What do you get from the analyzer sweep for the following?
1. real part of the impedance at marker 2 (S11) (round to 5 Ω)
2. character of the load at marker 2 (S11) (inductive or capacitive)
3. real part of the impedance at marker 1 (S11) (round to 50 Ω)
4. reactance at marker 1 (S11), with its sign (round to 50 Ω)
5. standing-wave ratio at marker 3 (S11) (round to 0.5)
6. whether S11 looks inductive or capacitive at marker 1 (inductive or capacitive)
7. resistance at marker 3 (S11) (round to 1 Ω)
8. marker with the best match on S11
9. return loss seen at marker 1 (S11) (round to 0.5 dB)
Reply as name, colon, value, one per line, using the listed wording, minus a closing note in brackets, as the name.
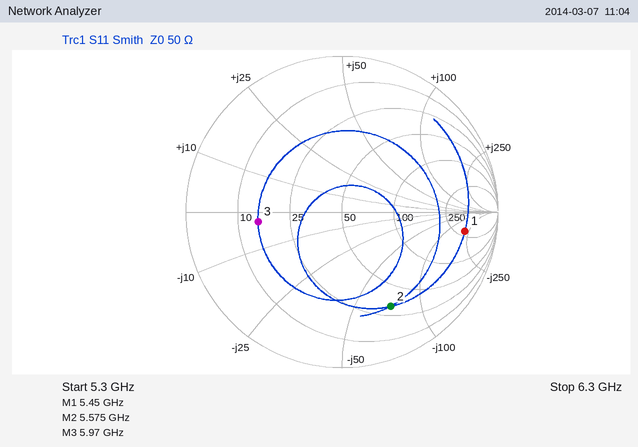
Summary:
real part of the impedance at marker 2 (S11): 30 Ω
character of the load at marker 2 (S11): capacitive
real part of the impedance at marker 1 (S11): 300 Ω
reactance at marker 1 (S11), with its sign: -200 Ω
standing-wave ratio at marker 3 (S11): 3.5
whether S11 looks inductive or capacitive at marker 1: capacitive
resistance at marker 3 (S11): 15 Ω
marker with the best match on S11: marker 3
return loss seen at marker 1 (S11): 2.0 dB
